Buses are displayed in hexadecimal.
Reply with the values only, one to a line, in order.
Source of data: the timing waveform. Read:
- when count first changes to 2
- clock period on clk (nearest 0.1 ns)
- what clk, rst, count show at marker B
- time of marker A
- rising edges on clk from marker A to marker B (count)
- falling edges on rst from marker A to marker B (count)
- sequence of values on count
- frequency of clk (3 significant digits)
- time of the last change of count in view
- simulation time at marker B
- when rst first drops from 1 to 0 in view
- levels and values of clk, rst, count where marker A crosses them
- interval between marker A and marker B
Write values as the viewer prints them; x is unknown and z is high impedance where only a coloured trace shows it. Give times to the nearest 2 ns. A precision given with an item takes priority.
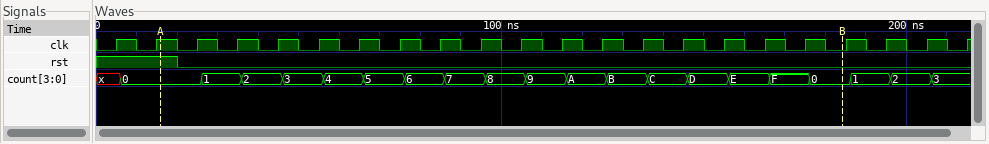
36 ns
10 ns
clk=0, rst=0, count=0
16 ns
16
1
x, 0, 1, 2, 3, 4, 5, 6, 7, 8, 9, A, B, C, D, E, F, 0, 1, 2, 3
100 MHz
206 ns
184 ns
20 ns
clk=1, rst=1, count=0
168 ns
